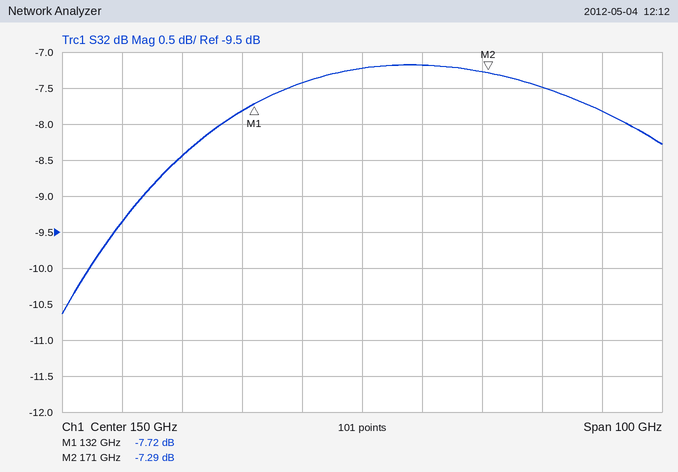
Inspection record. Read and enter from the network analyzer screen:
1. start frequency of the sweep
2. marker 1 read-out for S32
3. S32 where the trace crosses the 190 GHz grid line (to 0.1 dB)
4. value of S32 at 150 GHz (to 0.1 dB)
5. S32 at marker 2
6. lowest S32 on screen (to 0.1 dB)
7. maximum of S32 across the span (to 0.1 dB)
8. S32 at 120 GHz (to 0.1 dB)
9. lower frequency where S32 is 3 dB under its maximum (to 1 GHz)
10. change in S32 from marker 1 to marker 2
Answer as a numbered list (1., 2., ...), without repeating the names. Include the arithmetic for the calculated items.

1. 100 GHz
2. -7.72 dB
3. -7.8 dB
4. -7.2 dB
5. -7.29 dB
6. -10.6 dB
7. -7.2 dB
8. -8.4 dB
9. 103 GHz
10. -7.29 − (-7.72) = 0.43 dB
